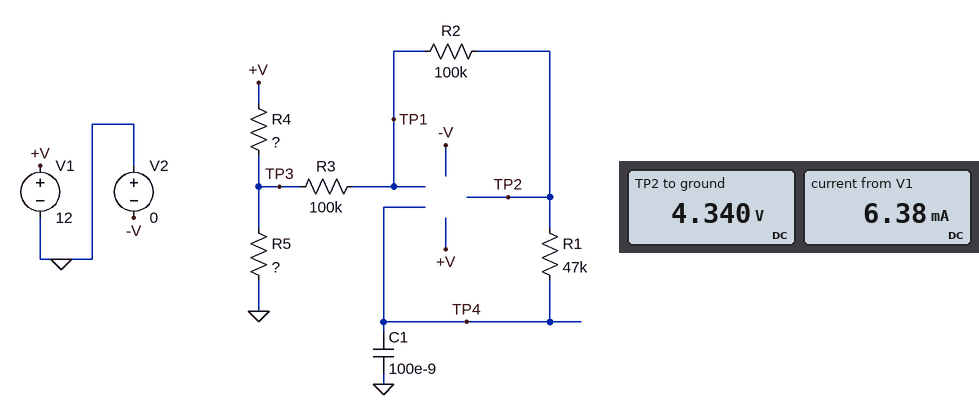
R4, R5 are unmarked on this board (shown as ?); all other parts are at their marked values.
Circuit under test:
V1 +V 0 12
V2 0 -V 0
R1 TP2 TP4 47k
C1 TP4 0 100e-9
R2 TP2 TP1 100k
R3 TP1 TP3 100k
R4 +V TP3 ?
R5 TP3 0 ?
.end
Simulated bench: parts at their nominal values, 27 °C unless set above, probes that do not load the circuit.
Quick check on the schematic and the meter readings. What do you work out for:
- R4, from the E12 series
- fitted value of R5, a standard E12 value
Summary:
1.2 kΩ
680 Ω
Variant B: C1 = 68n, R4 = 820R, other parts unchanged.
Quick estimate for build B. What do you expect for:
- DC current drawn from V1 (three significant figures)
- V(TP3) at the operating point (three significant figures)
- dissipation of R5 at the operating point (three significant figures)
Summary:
8.00 mA
5.44 V
43.5 mW
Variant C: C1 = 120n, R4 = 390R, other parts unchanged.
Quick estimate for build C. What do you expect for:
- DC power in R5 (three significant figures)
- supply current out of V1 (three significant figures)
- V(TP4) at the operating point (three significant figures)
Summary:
85.5 mW
11.2 mA
7.63 V
